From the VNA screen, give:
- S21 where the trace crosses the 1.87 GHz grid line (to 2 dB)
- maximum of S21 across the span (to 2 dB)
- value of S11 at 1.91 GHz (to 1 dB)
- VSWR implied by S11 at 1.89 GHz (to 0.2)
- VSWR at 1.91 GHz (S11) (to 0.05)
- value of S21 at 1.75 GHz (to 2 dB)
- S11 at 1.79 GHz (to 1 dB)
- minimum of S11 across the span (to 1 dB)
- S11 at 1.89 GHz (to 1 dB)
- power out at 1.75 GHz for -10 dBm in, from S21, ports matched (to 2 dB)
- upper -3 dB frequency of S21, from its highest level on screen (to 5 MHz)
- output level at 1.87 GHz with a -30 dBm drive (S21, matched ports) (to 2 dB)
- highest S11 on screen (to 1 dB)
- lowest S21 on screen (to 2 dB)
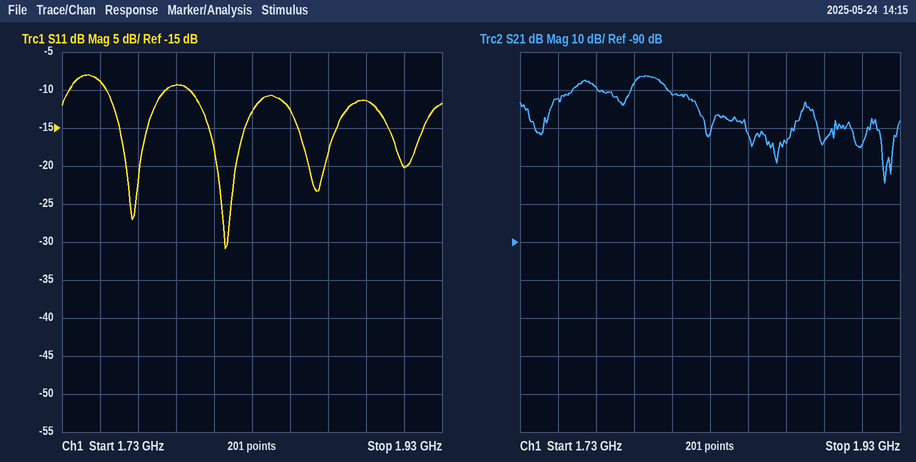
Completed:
-64 dB
-46 dB
-20 dB
1.8
1.20
-52 dB
-9 dB
-31 dB
-11 dB
-62 dBm
1.805 GHz
-94 dBm
-8 dB
-74 dB
